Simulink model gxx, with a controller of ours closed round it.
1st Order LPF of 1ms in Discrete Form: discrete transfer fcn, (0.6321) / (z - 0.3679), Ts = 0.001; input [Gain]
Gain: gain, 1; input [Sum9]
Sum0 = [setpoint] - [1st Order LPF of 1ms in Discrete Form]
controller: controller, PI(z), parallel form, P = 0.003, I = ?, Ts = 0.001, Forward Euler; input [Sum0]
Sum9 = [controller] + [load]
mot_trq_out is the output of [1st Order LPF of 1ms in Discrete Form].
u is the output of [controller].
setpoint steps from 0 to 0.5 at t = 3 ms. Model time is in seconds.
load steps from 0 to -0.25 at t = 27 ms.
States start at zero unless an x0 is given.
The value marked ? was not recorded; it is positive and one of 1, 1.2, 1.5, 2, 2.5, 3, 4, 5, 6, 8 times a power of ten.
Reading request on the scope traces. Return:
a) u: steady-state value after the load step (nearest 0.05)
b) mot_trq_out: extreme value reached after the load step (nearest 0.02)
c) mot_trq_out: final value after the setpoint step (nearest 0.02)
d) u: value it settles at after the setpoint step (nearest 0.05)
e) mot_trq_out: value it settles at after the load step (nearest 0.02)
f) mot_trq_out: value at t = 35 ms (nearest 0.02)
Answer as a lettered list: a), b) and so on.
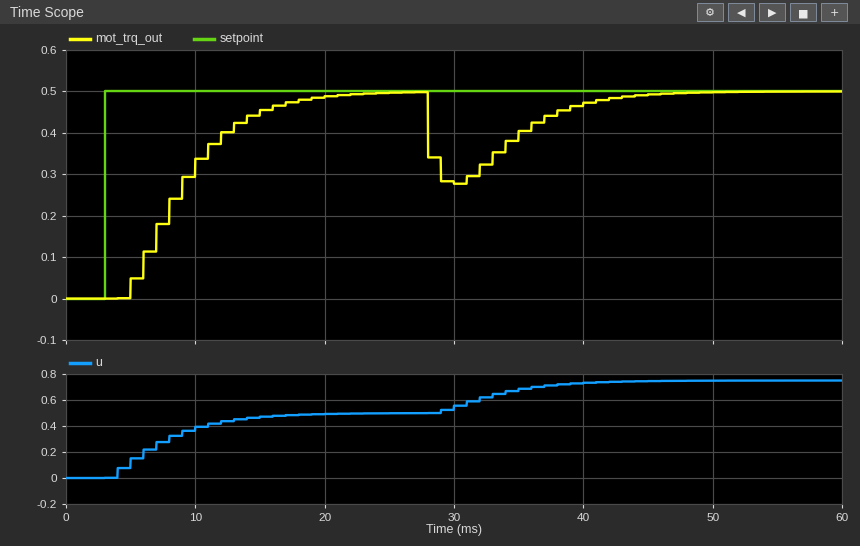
a) 0.75
b) 0.28
c) 0.50
d) 0.50
e) 0.50
f) 0.40
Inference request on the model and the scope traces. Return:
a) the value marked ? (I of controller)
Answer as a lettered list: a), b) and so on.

a) 150
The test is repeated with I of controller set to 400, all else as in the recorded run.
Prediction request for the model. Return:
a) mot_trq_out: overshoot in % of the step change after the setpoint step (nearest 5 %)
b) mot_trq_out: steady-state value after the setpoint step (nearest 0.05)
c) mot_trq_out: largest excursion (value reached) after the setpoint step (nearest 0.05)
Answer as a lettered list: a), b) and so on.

a) 25 %
b) 0.50
c) 0.60
